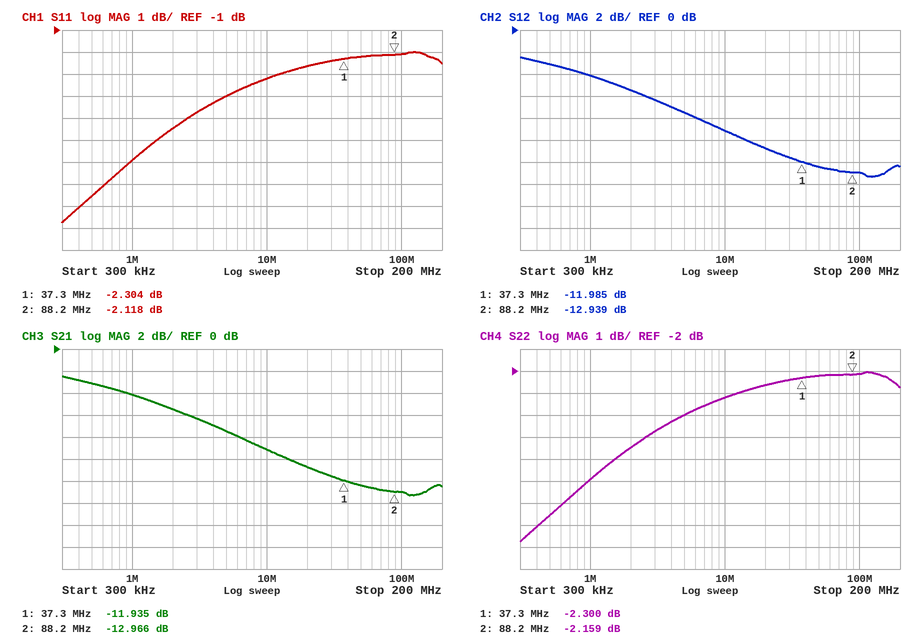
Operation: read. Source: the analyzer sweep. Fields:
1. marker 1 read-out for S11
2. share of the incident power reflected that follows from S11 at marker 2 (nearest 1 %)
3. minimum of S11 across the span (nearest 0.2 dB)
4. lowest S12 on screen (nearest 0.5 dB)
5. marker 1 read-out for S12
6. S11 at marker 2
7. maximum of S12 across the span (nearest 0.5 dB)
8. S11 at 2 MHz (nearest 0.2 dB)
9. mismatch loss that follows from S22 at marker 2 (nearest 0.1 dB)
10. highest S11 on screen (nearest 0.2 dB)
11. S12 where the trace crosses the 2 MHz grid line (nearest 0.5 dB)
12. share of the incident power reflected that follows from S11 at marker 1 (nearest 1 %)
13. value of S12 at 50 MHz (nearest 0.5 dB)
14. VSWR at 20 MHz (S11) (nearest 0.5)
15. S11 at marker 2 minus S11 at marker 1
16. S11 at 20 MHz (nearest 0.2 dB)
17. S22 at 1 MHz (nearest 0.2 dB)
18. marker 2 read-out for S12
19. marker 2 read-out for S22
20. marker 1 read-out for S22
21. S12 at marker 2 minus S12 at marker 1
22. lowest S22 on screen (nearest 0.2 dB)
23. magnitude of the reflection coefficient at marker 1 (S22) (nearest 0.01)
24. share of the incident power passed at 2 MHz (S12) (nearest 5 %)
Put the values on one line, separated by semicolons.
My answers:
-2.304 dB; 61 %; -9.8 dB; -13.5 dB; -11.985 dB; -2.118 dB; -2.5 dB; -5.4 dB; 4.1 dB; -2.0 dB; -5.5 dB; 59 %; -12.5 dB; 6.5; 0.186 dB; -2.6 dB; -7.0 dB; -12.939 dB; -2.159 dB; -2.300 dB; -0.954 dB; -9.8 dB; 0.77; 30 %
